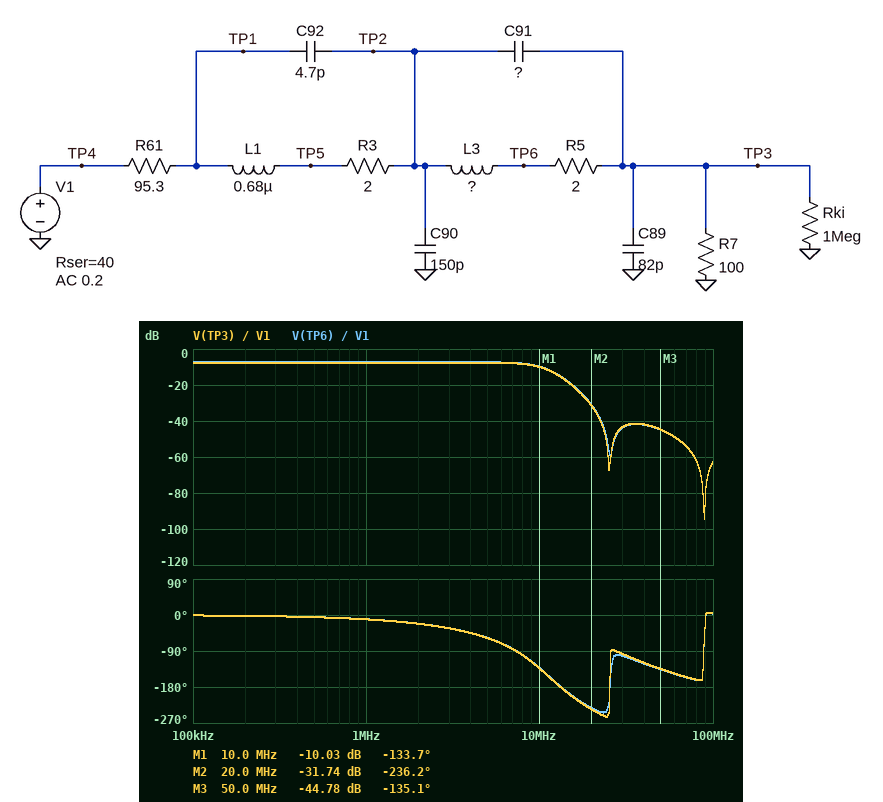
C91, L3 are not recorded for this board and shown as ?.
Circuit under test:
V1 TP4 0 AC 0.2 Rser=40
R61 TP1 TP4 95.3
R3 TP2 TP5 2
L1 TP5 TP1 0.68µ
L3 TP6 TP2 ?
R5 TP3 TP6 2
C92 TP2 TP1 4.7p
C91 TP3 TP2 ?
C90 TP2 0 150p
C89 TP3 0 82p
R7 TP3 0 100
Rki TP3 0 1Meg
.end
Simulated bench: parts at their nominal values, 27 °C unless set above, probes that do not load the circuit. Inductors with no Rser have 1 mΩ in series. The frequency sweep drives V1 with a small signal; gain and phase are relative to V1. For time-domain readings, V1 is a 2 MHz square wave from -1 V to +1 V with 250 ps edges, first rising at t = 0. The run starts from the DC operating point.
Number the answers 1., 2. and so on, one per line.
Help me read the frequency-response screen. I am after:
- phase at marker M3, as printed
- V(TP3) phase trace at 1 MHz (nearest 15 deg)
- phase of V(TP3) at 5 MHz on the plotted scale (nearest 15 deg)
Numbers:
1. -135.1 deg
2. -15 deg
3. -60 deg
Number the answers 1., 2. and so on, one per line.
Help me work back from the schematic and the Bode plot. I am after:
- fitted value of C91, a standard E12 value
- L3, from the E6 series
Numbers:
1. 12 pF
2. 3.3 µH
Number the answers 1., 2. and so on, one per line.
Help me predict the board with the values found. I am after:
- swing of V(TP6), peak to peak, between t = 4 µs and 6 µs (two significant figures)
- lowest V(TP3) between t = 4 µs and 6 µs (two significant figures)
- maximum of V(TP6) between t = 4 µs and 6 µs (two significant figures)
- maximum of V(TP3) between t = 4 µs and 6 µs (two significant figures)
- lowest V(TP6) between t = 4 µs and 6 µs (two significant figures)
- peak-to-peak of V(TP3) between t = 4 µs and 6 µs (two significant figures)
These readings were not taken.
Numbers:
1. 1.0 V
2. -500 mV
3. 510 mV
4. 500 mV
5. -510 mV
6. 1.0 V
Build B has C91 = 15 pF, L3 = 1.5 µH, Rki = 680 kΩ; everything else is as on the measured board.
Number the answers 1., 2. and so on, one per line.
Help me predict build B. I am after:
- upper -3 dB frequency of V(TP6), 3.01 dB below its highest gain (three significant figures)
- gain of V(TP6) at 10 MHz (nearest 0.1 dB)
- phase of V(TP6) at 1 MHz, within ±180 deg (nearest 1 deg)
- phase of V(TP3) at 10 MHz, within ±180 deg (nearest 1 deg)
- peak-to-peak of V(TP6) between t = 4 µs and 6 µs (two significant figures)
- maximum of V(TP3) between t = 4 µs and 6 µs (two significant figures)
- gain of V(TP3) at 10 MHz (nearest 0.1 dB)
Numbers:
1. 16.2 MHz
2. -7.4 dB
3. -8 deg
4. -88 deg
5. 1.1 V
6. 530 mV
7. -7.6 dB
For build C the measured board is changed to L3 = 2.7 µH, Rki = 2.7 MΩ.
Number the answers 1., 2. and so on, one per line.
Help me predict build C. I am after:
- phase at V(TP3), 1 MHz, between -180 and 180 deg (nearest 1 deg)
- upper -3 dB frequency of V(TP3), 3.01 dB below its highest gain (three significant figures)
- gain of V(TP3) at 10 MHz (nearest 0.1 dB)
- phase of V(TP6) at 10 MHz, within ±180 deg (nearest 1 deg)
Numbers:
1. -10 deg
2. 11.8 MHz
3. -8.6 dB
4. -120 deg
